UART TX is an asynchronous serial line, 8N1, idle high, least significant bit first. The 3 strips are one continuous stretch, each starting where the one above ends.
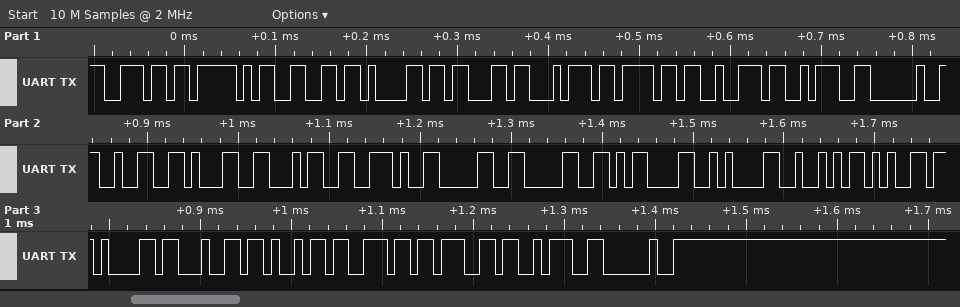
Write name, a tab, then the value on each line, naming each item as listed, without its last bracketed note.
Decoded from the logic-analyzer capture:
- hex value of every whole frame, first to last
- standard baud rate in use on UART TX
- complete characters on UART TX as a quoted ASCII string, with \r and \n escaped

hex value of every whole frame, first to last	6E 5F 66 61 63 74 6F 72 3A 20 32 31 34 2E 30 30 0D 0A 52 65 61 64 69 6E 67 3A 20
standard baud rate in use on UART TX	115200 baud
complete characters on UART TX as a quoted ASCII string, with \r and \n escaped	"n_factor: 214.00\r\nReading: "
